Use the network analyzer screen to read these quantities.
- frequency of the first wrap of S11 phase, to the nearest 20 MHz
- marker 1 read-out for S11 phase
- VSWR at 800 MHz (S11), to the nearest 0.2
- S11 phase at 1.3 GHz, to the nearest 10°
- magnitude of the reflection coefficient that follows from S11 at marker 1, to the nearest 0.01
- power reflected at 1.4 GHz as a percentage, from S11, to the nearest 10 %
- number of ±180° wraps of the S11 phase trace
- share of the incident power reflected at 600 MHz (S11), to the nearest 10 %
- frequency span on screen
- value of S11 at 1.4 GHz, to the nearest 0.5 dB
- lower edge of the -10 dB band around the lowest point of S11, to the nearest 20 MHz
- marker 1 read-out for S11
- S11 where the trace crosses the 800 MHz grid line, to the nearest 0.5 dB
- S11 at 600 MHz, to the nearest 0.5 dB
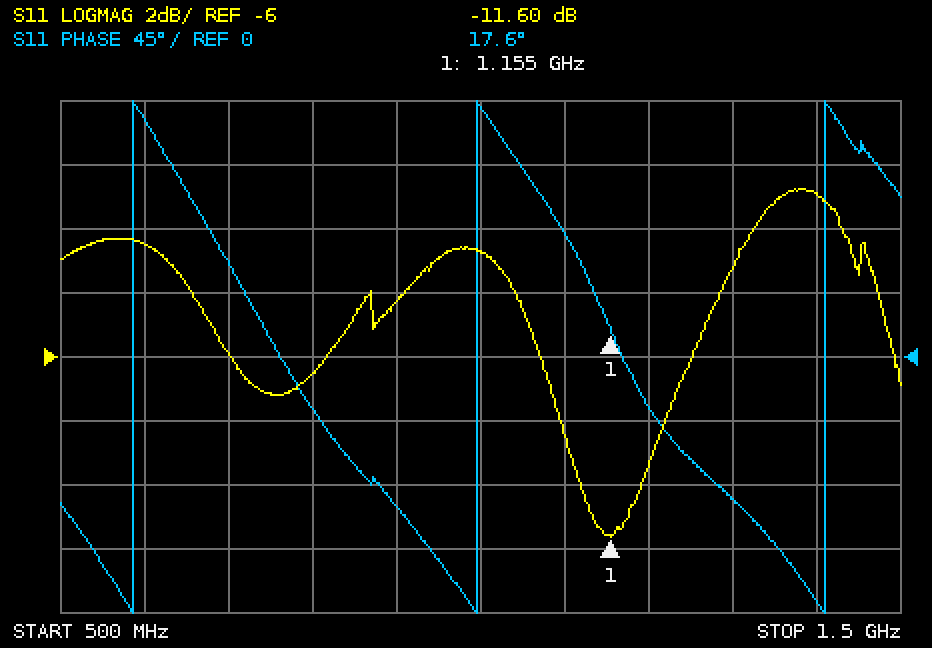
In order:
580 MHz
17.6°
2.8
-100°
0.26
80 %
3
60 %
1 GHz
-1.0 dB
1.12 GHz
-11.60 dB
-6.5 dB
-2.5 dB
